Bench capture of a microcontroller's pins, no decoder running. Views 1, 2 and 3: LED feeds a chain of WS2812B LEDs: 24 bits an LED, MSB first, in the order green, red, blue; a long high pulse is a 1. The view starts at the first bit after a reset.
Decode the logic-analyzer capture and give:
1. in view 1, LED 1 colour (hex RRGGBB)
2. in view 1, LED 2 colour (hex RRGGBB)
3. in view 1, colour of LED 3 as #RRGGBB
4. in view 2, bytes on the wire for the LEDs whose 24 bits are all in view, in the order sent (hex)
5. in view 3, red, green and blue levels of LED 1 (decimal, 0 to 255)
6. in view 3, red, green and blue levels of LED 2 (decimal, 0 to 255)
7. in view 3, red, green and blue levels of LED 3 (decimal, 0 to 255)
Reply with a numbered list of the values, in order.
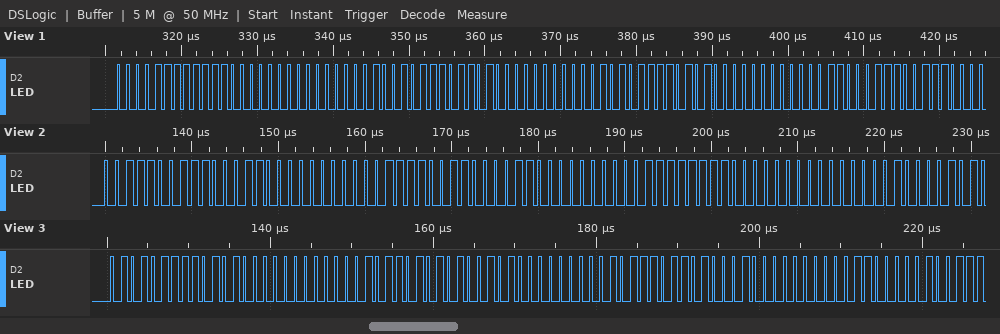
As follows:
1. #F00F00
2. #ED1200
3. #EA1500
4. 39 C6 00 3C C3 00 3F C0 00
5. 168, 87, 0
6. 165, 90, 0
7. 162, 93, 0
